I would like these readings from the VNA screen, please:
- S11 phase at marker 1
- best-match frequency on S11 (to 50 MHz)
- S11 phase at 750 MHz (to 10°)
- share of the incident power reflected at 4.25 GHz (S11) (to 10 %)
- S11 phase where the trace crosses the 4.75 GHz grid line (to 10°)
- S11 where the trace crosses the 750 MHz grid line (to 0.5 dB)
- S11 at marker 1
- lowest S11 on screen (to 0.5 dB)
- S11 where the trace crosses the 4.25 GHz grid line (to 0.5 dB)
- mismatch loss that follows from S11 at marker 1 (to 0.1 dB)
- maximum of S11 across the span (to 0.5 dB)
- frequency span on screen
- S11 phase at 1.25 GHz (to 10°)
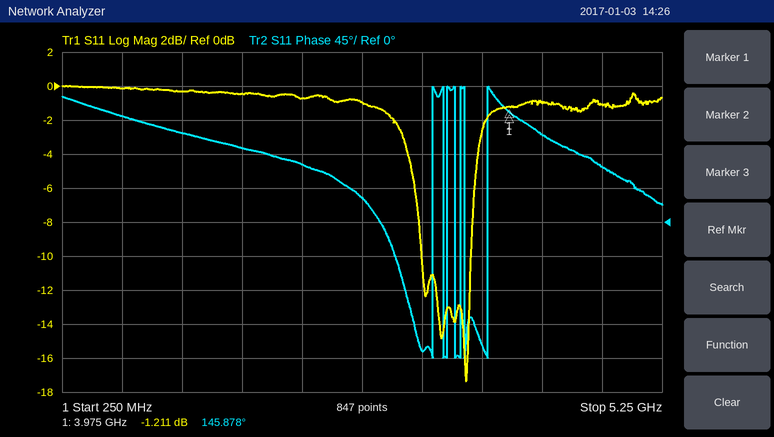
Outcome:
145.878°
3.60 GHz
140°
80 %
70°
0.0 dB
-1.211 dB
-17.5 dB
-1.0 dB
6.1 dB
0.0 dB
5 GHz
120°
